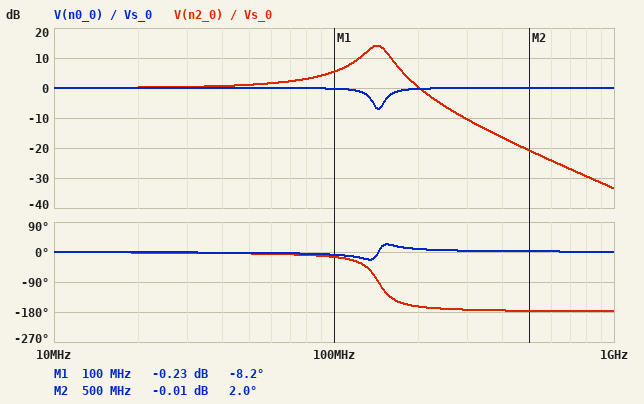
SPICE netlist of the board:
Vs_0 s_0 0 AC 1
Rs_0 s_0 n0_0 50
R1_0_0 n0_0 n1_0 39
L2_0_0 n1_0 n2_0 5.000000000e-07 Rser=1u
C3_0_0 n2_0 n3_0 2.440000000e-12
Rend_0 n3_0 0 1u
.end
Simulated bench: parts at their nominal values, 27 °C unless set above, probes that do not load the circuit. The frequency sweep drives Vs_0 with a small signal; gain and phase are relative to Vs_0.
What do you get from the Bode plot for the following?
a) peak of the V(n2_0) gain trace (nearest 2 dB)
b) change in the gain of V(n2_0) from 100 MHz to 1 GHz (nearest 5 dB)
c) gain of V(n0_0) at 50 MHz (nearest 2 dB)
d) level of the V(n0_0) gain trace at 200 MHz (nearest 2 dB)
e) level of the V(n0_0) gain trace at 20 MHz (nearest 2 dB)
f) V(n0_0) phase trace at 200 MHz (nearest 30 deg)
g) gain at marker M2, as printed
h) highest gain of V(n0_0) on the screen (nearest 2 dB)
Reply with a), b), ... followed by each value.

a) 14 dB
b) -40 dB
c) 0 dB
d) 0 dB
e) 0 dB
f) 0 deg
g) -0.01 dB
h) 0 dB
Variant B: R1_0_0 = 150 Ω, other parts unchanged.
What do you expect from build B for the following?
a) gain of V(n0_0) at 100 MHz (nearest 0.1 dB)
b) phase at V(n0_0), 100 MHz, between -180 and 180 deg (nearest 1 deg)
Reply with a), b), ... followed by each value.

a) -0.5 dB
b) -7 deg
